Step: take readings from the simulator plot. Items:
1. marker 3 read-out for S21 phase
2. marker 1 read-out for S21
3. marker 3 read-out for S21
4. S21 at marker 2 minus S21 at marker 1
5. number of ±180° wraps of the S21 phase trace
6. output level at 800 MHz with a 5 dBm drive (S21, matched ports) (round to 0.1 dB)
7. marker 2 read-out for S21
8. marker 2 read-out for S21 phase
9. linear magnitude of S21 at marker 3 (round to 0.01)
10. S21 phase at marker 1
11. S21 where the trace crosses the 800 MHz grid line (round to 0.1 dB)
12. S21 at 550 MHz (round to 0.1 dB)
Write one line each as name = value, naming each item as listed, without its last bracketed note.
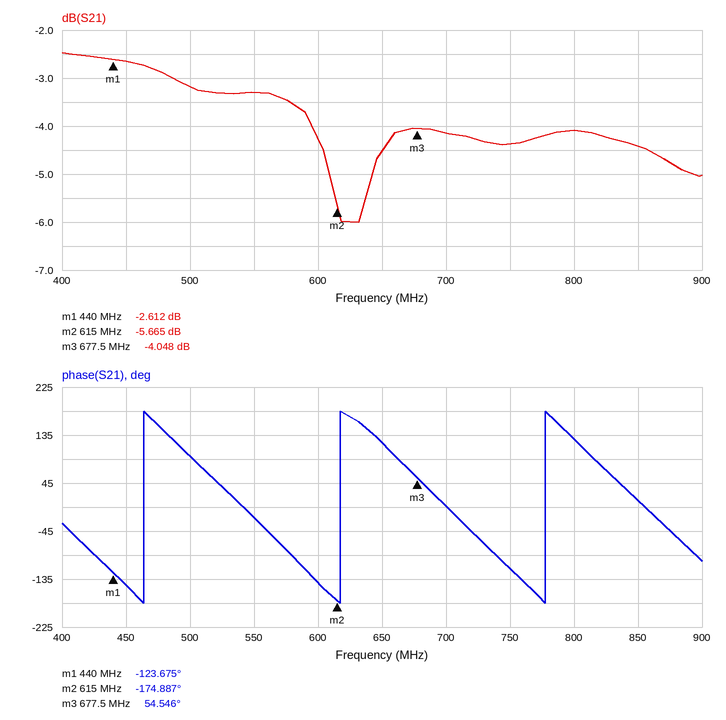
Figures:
marker 3 read-out for S21 phase = 54.546°
marker 1 read-out for S21 = -2.612 dB
marker 3 read-out for S21 = -4.048 dB
S21 at marker 2 minus S21 at marker 1 = -3.053 dB
number of ±180° wraps of the S21 phase trace = 3
output level at 800 MHz with a 5 dBm drive (S21, matched ports) = 0.9 dBm
marker 2 read-out for S21 = -5.665 dB
marker 2 read-out for S21 phase = -174.887°
linear magnitude of S21 at marker 3 = 0.63
S21 phase at marker 1 = -123.675°
S21 where the trace crosses the 800 MHz grid line = -4.1 dB
S21 at 550 MHz = -3.3 dB
